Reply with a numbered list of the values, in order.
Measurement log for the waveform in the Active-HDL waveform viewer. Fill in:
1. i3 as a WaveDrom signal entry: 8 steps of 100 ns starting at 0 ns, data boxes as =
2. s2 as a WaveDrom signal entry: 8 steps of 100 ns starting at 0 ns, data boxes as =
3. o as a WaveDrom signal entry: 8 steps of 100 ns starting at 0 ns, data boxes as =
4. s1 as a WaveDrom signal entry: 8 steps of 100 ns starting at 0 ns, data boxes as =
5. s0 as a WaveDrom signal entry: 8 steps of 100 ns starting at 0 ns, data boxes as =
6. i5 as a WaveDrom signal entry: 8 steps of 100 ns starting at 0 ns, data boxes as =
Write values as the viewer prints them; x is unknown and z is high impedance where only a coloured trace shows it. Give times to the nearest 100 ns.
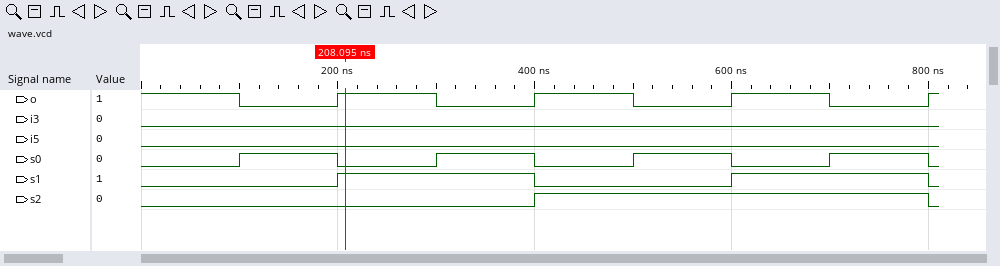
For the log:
1. {name: 'i3', wave: '0.......'}
2. {name: 's2', wave: '0...1...'}
3. {name: 'o', wave: '10101010'}
4. {name: 's1', wave: '0.1.0.1.'}
5. {name: 's0', wave: '01010101'}
6. {name: 'i5', wave: '0.......'}
